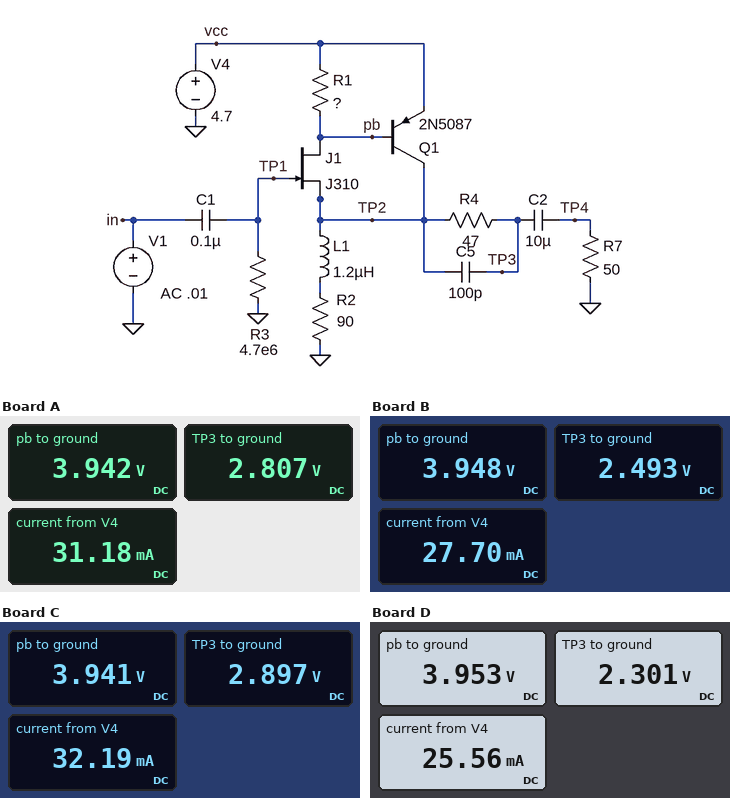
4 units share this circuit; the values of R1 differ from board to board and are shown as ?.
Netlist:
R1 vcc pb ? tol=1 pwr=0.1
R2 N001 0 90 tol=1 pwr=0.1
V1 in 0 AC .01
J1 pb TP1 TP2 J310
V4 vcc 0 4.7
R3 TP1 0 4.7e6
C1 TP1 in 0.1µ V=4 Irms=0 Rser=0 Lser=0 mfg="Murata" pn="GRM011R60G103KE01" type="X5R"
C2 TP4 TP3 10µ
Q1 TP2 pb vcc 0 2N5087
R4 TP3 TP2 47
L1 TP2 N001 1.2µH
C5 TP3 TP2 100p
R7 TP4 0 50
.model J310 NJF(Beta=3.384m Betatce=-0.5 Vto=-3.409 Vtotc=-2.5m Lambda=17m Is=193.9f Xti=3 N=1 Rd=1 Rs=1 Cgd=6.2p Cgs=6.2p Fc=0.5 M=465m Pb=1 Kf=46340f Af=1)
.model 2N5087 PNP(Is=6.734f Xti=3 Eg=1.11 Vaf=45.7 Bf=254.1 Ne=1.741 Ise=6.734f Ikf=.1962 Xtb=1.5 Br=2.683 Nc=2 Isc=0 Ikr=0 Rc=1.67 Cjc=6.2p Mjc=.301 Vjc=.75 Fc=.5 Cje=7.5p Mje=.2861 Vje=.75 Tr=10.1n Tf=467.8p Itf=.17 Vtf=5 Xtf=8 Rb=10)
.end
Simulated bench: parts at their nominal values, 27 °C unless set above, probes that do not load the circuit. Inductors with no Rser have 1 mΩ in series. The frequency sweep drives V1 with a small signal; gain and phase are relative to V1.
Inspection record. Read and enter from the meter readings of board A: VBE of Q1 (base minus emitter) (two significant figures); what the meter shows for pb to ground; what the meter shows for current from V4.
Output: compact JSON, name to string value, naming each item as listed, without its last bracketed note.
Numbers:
{"VBE of Q1 (base minus emitter)": "-760 mV", "what the meter shows for pb to ground": "3.942 V", "what the meter shows for current from V4": "31.18 mA"}
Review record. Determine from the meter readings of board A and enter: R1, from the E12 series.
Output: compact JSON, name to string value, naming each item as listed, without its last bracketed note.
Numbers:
{"R1, from the E12 series": "680 Ω"}
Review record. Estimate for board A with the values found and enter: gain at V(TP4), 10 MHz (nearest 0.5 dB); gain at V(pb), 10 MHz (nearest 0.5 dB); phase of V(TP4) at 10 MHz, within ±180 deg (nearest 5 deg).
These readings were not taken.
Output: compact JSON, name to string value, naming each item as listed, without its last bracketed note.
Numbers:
{"gain at V(TP4), 10 MHz": "-6.5 dB", "gain at V(pb), 10 MHz": "-34.5 dB", "phase of V(TP4) at 10 MHz, within ±180 deg": "-10 deg"}
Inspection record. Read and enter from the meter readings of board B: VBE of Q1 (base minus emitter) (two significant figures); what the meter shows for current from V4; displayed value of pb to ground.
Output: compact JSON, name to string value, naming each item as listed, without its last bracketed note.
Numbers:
{"VBE of Q1 (base minus emitter)": "-750 mV", "what the meter shows for current from V4": "27.70 mA", "displayed value of pb to ground": "3.948 V"}
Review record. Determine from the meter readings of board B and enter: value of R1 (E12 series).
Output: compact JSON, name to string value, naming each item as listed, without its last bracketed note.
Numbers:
{"value of R1": "270 Ω"}
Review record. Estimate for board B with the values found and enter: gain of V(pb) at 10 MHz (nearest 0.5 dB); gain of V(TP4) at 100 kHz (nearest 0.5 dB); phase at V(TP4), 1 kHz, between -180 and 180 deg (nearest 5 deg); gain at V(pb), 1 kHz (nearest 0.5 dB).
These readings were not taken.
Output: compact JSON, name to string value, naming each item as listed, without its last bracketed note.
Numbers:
{"gain of V(pb) at 10 MHz": "-33.5 dB", "gain of V(TP4) at 100 kHz": "-6.0 dB", "phase at V(TP4), 1 kHz, between -180 and 180 deg": "10 deg", "gain at V(pb), 1 kHz": "-32.0 dB"}
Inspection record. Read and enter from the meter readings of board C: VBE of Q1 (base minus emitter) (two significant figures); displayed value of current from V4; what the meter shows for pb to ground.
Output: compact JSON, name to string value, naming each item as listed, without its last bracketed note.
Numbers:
{"VBE of Q1 (base minus emitter)": "-760 mV", "displayed value of current from V4": "32.19 mA", "what the meter shows for pb to ground": "3.941 V"}
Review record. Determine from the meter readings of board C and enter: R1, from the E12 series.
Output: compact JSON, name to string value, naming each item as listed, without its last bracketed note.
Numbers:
{"R1, from the E12 series": "1 kΩ"}
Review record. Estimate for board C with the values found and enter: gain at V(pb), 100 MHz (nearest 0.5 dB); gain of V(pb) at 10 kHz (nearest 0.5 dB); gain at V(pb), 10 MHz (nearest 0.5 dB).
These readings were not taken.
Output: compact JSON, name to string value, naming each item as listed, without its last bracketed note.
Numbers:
{"gain at V(pb), 100 MHz": "-28.5 dB", "gain of V(pb) at 10 kHz": "-33.5 dB", "gain at V(pb), 10 MHz": "-35.0 dB"}
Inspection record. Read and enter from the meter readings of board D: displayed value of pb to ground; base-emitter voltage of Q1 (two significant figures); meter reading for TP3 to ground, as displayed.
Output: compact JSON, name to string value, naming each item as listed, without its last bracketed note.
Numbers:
{"displayed value of pb to ground": "3.953 V", "base-emitter voltage of Q1": "-750 mV", "meter reading for TP3 to ground, as displayed": "2.301 V"}
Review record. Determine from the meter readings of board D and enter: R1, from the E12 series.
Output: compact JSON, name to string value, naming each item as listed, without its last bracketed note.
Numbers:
{"R1, from the E12 series": "180 Ω"}
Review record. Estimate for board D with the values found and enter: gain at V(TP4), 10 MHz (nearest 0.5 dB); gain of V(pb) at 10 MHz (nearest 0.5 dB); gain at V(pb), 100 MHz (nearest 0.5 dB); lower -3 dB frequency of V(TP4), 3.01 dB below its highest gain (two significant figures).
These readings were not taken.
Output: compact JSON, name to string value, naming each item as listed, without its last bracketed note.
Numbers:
{"gain at V(TP4), 10 MHz": "-6.0 dB", "gain of V(pb) at 10 MHz": "-32.5 dB", "gain at V(pb), 100 MHz": "-25.0 dB", "lower -3 dB frequency of V(TP4), 3.01 dB below its highest gain": "260 Hz"}
